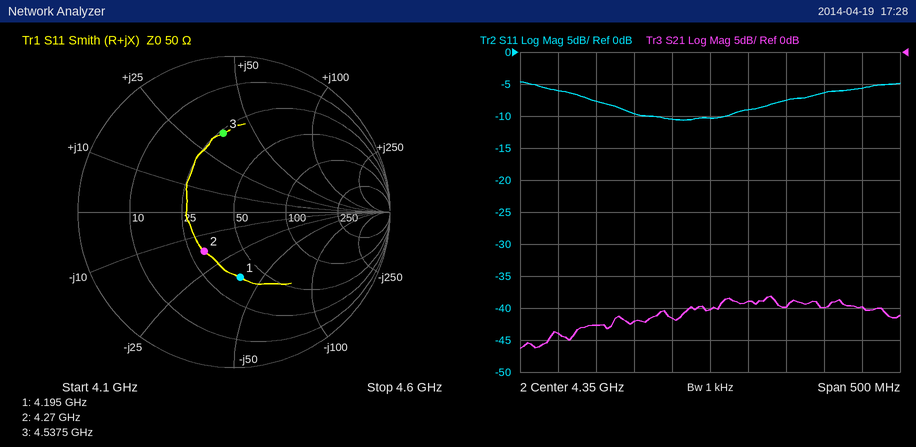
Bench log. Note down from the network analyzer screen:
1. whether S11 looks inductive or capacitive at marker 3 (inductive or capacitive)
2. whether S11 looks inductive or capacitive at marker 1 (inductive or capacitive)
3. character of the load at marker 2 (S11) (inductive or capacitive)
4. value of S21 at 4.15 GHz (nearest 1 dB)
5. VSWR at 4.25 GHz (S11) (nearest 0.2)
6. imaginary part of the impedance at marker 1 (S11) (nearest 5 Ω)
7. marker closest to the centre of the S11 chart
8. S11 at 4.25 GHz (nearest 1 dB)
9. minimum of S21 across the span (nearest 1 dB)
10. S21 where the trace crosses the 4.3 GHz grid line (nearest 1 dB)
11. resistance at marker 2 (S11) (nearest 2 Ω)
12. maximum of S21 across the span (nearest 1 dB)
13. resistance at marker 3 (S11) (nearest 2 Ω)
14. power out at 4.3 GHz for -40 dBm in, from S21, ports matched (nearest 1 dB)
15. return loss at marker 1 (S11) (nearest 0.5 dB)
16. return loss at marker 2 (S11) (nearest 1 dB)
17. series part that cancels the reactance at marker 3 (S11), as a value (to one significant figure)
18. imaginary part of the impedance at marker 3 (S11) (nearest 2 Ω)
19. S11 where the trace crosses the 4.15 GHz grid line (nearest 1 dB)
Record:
inductive
capacitive
capacitive
-44 dB
2.0
-40 Ω
marker 2
-10 dB
-46 dB
-42 dB
30 Ω
-38 dB
26 Ω
-82 dBm
7.5 dB
10 dB
1.0 pF
+36 Ω
-6 dB
